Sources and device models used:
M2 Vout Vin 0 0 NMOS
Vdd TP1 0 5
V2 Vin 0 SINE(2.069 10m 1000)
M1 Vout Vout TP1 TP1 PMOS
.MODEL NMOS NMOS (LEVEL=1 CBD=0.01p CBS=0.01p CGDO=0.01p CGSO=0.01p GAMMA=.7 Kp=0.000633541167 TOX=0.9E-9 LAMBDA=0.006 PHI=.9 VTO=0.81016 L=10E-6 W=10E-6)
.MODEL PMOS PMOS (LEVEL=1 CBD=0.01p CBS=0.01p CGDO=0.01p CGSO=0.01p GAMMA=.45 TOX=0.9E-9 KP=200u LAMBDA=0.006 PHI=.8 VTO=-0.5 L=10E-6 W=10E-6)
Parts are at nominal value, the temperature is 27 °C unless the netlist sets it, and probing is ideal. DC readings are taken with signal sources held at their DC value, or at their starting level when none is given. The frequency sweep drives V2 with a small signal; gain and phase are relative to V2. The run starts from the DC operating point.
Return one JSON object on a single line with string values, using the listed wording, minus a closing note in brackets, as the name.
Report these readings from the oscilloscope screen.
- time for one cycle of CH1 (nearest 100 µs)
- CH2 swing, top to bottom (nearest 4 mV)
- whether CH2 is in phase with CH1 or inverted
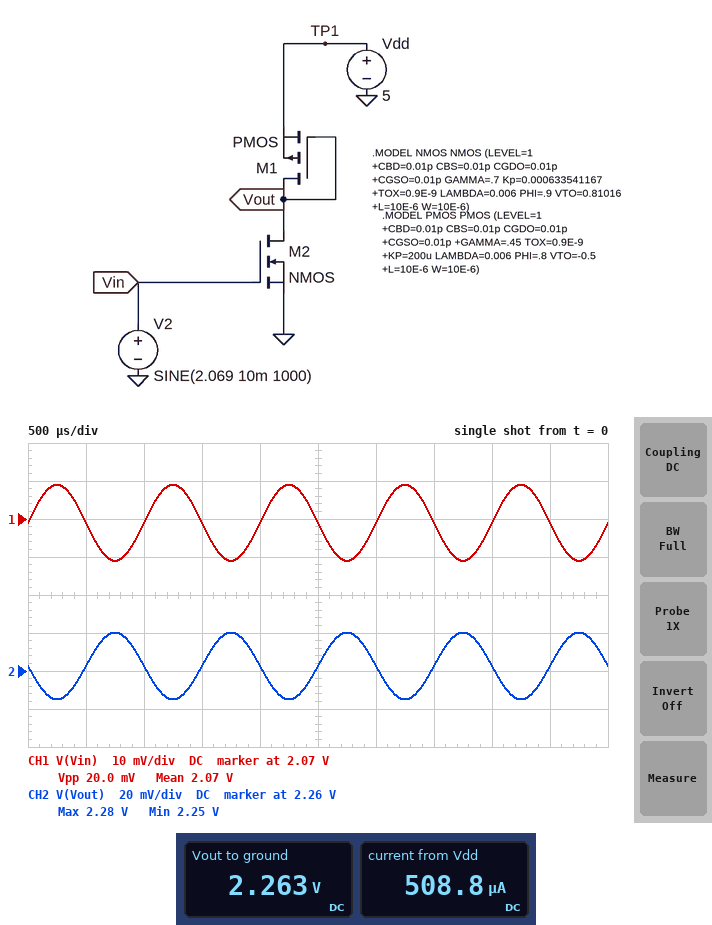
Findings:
{"time for one cycle of CH1": "1.0 ms", "CH2 swing, top to bottom": "36 mV", "whether CH2 is in phase with CH1 or inverted": "inverted"}
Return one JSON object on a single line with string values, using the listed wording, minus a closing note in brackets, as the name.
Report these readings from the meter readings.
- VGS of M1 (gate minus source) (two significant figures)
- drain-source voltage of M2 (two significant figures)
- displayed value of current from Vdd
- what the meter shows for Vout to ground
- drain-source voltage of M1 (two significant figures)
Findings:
{"VGS of M1 (gate minus source)": "-2.7 V", "drain-source voltage of M2": "2.3 V", "displayed value of current from Vdd": "508.8 µA", "what the meter shows for Vout to ground": "2.263 V", "drain-source voltage of M1": "-2.7 V"}
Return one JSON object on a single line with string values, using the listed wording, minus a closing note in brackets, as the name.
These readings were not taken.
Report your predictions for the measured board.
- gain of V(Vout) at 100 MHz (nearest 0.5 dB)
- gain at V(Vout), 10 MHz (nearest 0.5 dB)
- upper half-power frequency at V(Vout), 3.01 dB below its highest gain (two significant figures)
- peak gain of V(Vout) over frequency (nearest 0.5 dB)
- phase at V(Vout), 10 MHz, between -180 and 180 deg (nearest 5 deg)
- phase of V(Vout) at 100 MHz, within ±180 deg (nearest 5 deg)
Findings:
{"gain of V(Vout) at 100 MHz": "-6.5 dB", "gain at V(Vout), 10 MHz": "4.5 dB", "upper half-power frequency at V(Vout), 3.01 dB below its highest gain": "29 MHz", "peak gain of V(Vout) over frequency": "5.0 dB", "phase at V(Vout), 10 MHz, between -180 and 180 deg": "160 deg", "phase of V(Vout) at 100 MHz, within ±180 deg": "105 deg"}
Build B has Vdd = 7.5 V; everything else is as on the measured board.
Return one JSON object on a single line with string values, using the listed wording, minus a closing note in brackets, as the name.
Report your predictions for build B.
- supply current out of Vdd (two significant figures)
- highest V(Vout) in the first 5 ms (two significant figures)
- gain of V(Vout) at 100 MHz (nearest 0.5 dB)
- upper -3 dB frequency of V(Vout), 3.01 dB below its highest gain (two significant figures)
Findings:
{"supply current out of Vdd": "520 µA", "highest V(Vout) in the first 5 ms": "4.8 V", "gain of V(Vout) at 100 MHz": "-6.0 dB", "upper -3 dB frequency of V(Vout), 3.01 dB below its highest gain": "29 MHz"}
